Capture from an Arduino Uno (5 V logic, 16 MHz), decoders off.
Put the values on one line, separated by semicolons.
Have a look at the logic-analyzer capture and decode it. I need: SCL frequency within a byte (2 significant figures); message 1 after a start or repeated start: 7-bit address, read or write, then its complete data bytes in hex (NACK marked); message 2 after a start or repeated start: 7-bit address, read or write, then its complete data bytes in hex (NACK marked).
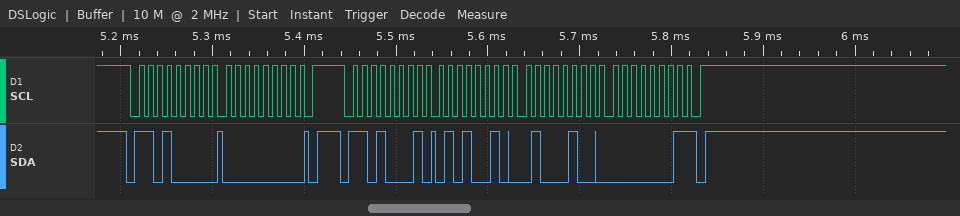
100 kHz; 0x68 write: 00; 0x68 read: 52 44 01 NACK
